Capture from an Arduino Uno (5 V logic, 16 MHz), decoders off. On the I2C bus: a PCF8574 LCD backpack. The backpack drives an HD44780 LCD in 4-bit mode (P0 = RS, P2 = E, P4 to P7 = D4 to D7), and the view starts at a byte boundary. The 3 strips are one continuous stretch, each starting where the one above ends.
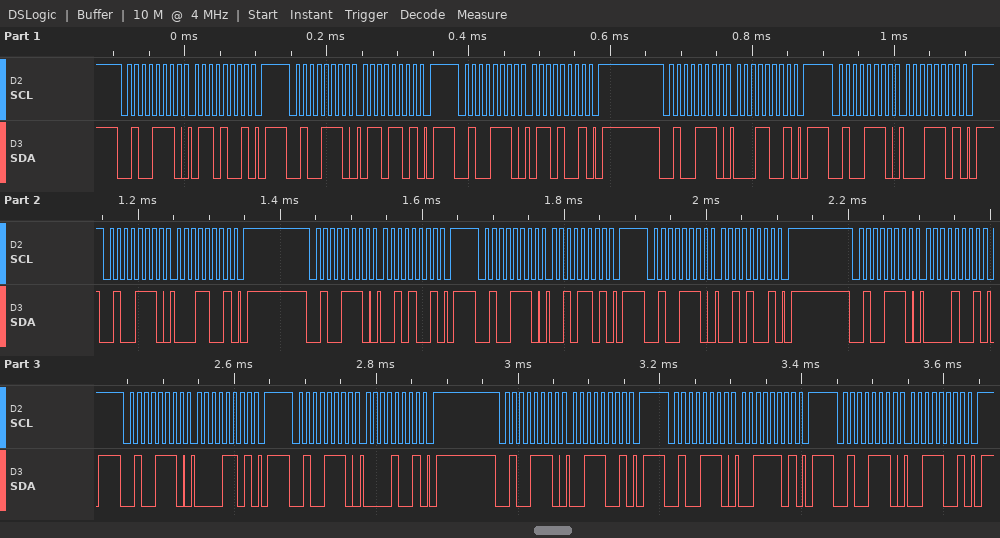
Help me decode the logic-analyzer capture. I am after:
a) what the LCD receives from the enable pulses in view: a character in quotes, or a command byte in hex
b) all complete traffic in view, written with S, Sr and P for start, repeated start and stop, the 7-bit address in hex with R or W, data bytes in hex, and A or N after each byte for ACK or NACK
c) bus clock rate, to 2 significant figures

'a' ' '
S 27W A 69 A P S 27W A 6D A P S 27W A 69 A P S 27W A 19 A P S 27W A 1D A P S 27W A 19 A P S 27W A 29 A P S 27W A 2D A P S 27W A 29 A P S 27W A 09 A P S 27W A 0D A P S 27W A 09 A P S 27W A 39 A P S 27W A 3D A P S 27W A 39 A P
100 kHz
